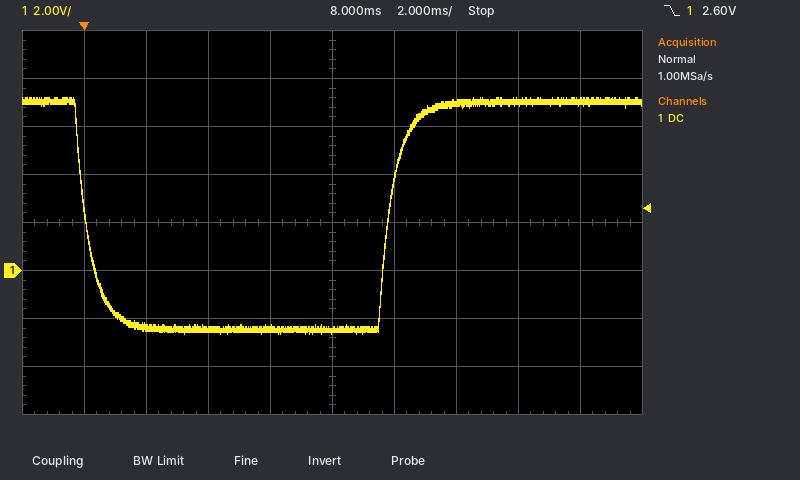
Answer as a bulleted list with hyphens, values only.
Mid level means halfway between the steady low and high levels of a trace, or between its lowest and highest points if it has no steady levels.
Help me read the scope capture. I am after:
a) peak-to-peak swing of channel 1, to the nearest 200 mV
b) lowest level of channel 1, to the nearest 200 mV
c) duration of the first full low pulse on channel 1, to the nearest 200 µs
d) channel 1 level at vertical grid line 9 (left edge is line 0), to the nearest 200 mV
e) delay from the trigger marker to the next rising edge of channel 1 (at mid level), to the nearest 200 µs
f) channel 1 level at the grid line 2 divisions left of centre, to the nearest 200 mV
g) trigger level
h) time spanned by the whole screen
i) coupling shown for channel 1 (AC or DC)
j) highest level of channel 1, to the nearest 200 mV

- 9.8 V
- -2.6 V
- 9.8 ms
- 7.0 V
- 9.8 ms
- -2.4 V
- 2.60 V
- 20 ms
- DC
- 7.2 V
